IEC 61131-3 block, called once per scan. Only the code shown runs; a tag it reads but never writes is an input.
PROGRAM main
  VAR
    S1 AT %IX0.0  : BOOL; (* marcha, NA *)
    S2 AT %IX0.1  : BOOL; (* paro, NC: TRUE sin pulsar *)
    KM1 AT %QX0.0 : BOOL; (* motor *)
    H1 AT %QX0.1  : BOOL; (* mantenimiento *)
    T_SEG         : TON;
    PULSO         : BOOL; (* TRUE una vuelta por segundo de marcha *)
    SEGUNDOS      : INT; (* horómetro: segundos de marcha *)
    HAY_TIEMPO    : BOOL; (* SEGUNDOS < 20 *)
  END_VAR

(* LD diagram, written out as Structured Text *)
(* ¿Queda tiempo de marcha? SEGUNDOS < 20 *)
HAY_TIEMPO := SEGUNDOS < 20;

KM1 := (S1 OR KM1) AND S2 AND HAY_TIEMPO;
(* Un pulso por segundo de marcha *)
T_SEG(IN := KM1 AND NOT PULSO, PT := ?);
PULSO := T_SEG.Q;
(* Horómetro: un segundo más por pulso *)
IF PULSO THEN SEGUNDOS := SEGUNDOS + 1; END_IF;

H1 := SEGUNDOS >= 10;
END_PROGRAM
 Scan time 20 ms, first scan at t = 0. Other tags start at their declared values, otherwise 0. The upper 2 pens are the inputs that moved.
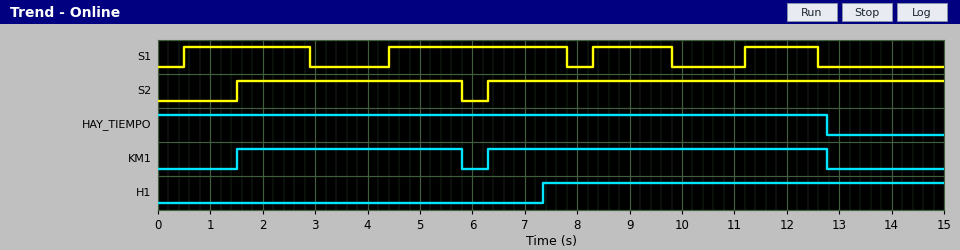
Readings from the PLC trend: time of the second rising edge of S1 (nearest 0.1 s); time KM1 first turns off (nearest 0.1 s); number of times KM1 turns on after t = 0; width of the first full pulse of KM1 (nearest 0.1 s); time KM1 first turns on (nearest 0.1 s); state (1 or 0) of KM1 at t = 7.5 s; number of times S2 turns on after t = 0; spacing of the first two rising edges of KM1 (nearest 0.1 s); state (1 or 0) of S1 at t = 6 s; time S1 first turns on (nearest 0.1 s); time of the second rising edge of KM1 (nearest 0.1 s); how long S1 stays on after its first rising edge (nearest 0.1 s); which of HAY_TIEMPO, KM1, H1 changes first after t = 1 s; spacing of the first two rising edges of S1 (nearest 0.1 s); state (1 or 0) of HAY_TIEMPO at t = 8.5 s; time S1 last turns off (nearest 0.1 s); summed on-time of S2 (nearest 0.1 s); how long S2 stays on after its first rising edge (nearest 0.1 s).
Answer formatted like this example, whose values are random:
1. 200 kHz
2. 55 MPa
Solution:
1. 4.4 s
2. 5.8 s
3. 2
4. 4.3 s
5. 1.5 s
6. 1
7. 2
8. 4.8 s
9. 1
10. 0.5 s
11. 6.3 s
12. 2.4 s
13. KM1
14. 3.9 s
15. 1
16. 12.6 s
17. 13.0 s
18. 4.3 s
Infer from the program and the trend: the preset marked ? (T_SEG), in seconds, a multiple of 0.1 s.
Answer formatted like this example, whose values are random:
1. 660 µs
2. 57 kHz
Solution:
1. 0.5 s
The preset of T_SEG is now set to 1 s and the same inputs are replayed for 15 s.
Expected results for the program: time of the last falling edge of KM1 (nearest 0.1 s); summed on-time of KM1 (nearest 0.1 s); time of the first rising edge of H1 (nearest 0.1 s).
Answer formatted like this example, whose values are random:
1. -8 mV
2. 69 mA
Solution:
1. 5.8 s
2. 13.0 s
3. 12.5 s
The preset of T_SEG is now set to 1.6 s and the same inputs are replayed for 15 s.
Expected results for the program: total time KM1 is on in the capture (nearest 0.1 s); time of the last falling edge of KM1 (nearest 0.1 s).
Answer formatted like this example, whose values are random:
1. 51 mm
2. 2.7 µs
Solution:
1. 13.0 s
2. 5.8 s
